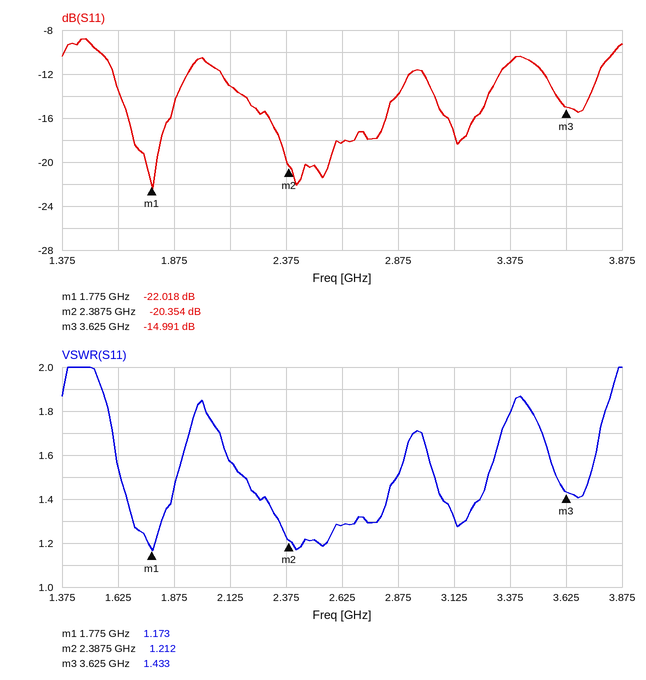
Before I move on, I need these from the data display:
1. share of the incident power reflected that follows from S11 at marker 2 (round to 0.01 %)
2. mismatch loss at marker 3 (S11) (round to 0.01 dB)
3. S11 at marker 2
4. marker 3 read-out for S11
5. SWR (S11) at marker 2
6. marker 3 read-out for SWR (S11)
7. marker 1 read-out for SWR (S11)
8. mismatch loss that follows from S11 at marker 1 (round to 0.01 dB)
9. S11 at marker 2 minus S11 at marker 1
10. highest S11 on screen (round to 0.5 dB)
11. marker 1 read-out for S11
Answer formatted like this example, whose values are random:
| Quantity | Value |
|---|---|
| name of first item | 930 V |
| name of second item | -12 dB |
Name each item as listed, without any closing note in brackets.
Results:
| Quantity | Value |
|---|---|
| share of the incident power reflected that follows from S11 at marker 2 | 0.92 % |
| mismatch loss at marker 3 (S11) | 0.14 dB |
| S11 at marker 2 | -20.354 dB |
| marker 3 read-out for S11 | -14.991 dB |
| SWR (S11) at marker 2 | 1.212 |
| marker 3 read-out for SWR | 1.433 |
| marker 1 read-out for SWR | 1.173 |
| mismatch loss that follows from S11 at marker 1 | 0.03 dB |
| S11 at marker 2 minus S11 at marker 1 | 1.664 dB |
| highest S11 on screen | -9.0 dB |
| marker 1 read-out for S11 | -22.018 dB |
